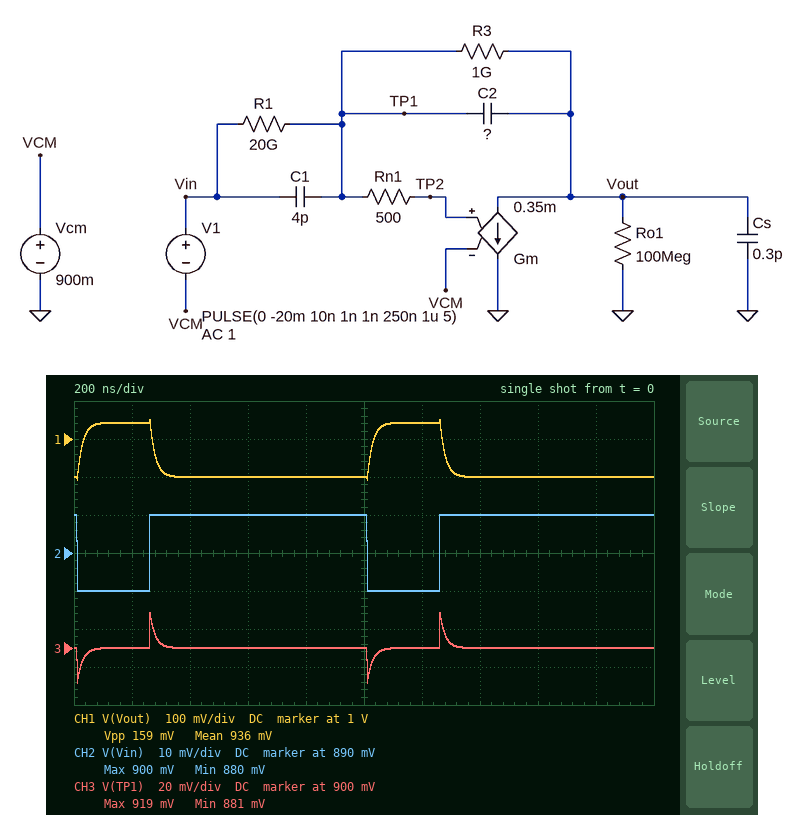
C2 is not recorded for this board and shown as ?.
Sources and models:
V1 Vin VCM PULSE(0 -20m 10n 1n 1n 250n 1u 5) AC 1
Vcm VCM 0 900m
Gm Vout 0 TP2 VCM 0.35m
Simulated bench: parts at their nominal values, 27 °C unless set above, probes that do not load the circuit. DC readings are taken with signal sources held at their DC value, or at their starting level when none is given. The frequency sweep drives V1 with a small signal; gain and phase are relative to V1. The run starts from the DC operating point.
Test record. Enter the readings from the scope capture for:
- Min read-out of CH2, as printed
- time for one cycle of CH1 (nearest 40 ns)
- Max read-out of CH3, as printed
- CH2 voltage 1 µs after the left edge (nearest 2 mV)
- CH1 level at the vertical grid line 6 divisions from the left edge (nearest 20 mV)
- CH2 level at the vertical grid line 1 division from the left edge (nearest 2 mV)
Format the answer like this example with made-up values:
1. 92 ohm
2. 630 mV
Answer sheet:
1. 880 mV
2. 1.00 µs
3. 919 mV
4. 900 mV
5. 1.04 V
6. 880 mV
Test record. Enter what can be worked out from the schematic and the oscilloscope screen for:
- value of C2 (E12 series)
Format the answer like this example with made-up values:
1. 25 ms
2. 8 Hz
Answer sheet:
1. 560 fF
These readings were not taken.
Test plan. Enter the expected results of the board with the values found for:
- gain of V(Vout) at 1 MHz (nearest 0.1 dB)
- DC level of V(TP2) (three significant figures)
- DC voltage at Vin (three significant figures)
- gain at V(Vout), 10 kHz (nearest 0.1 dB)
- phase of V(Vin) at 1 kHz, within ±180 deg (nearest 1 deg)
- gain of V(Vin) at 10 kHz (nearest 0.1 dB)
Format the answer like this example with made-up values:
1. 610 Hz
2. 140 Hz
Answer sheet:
1. 17.0 dB
2. 900 mV
3. 900 mV
4. 17.1 dB
5. 0 deg
6. 0 dB
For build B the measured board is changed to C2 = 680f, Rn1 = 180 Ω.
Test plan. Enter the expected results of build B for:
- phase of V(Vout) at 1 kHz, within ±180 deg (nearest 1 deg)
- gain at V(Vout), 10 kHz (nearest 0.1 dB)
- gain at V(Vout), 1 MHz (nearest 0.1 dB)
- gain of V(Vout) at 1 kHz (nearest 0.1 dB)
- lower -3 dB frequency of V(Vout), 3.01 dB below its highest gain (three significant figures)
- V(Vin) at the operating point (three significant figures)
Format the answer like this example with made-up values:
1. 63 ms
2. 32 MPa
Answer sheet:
1. -167 deg
2. 15.4 dB
3. 15.3 dB
4. 15.2 dB
5. 234 Hz
6. 900 mV
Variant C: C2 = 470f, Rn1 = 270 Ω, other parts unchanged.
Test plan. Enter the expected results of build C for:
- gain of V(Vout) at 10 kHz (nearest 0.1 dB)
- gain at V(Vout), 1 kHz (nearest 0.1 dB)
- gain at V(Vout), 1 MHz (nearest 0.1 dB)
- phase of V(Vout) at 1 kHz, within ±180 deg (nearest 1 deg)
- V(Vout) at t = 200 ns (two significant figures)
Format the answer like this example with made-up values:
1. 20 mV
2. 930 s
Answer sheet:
1. 18.6 dB
2. 18.1 dB
3. 18.5 dB
4. -161 deg
5. 1.1 V
